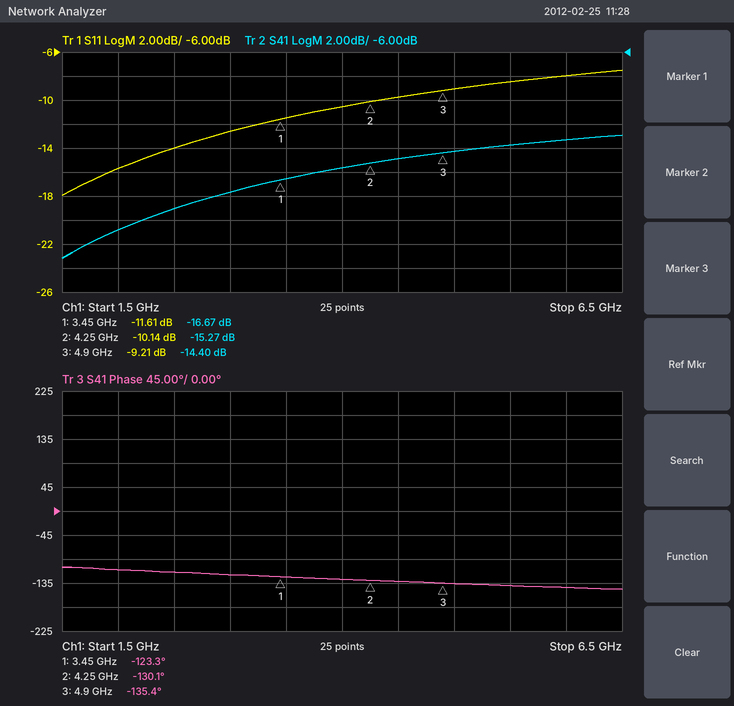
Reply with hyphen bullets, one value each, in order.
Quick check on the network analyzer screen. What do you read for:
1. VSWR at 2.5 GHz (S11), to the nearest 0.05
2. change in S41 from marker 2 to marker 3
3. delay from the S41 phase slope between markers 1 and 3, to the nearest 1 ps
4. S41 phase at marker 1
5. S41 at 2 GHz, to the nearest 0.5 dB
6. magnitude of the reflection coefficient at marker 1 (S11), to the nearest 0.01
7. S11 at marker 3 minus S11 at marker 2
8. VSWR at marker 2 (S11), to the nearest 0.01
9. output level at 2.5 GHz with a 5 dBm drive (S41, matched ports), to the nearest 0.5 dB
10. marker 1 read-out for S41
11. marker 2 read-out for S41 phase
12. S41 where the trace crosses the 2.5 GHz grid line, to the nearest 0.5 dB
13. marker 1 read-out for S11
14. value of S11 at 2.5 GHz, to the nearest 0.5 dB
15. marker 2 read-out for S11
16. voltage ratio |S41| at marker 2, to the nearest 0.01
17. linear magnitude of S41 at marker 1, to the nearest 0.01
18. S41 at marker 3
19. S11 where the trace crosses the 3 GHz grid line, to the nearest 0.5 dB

- 1.50
- 0.87 dB
- 23 ps
- -123.3°
- -21.0 dB
- 0.26
- 0.93 dB
- 1.90
- -14.0 dBm
- -16.67 dB
- -130.1°
- -19.0 dB
- -11.61 dB
- -14.0 dB
- -10.14 dB
- 0.17
- 0.15
- -14.40 dB
- -12.5 dB
